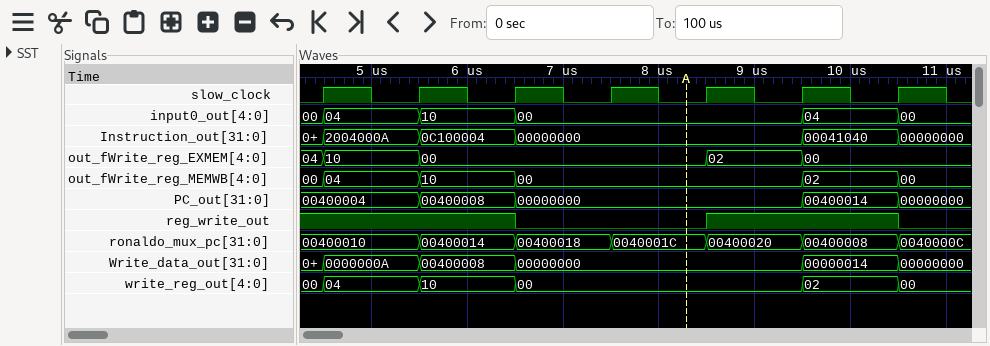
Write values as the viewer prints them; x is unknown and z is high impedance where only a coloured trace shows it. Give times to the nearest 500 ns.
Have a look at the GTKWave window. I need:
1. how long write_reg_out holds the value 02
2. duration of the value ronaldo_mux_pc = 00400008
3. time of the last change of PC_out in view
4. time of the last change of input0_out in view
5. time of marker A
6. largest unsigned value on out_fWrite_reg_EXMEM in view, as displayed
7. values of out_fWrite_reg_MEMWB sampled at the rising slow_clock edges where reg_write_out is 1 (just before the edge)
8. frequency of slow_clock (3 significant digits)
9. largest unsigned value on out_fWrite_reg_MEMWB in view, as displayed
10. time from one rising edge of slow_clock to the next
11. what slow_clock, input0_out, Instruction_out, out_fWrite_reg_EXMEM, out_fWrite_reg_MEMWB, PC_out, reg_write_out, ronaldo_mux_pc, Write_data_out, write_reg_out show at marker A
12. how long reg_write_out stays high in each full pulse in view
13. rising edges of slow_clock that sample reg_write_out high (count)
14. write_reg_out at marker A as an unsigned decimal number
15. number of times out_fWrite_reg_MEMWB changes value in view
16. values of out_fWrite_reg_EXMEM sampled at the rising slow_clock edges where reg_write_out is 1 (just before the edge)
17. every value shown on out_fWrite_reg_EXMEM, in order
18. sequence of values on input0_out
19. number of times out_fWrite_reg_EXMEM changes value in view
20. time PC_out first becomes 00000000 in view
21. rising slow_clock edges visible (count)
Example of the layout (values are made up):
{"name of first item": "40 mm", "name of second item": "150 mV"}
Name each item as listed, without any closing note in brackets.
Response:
{"how long write_reg_out holds the value 02": "1000 ns", "duration of the value ronaldo_mux_pc = 00400008": "1000 ns", "time of the last change of PC_out in view": "10500 ns", "time of the last change of input0_out in view": "10500 ns", "time of marker A": "8500 ns", "largest unsigned value on out_fWrite_reg_EXMEM in view, as displayed": "10", "values of out_fWrite_reg_MEMWB sampled at the rising slow_clock edges where reg_write_out is 1": "00, 04, 10, 00, 02", "frequency of slow_clock": "1.00 MHz", "largest unsigned value on out_fWrite_reg_MEMWB in view, as displayed": "10", "time from one rising edge of slow_clock to the next": "1000 ns", "what slow_clock, input0_out, Instruction_out, out_fWrite_reg_EXMEM, out_fWrite_reg_MEMWB, PC_out, reg_write_out, ronaldo_mux_pc, Write_data_out, write_reg_out show at marker A": "slow_clock=0, input0_out=00, Instruction_out=00000000, out_fWrite_reg_EXMEM=00, out_fWrite_reg_MEMWB=00, PC_out=00000000, reg_write_out=0, ronaldo_mux_pc=0040001C, Write_data_out=00000000, write_reg_out=00", "how long reg_write_out stays high in each full pulse in view": "2000 ns", "rising edges of slow_clock that sample reg_write_out high": "5", "write_reg_out at marker A as an unsigned decimal number": "0", "number of times out_fWrite_reg_MEMWB changes value in view": "5", "values of out_fWrite_reg_EXMEM sampled at the rising slow_clock edges where reg_write_out is 1": "04, 10, 00, 02, 00", "every value shown on out_fWrite_reg_EXMEM, in order": "04, 10, 00, 02, 00", "sequence of values on input0_out": "00, 04, 10, 00, 04, 00", "number of times out_fWrite_reg_EXMEM changes value in view": "4", "time PC_out first becomes 00000000 in view": "6500 ns", "rising slow_clock edges visible": "7"}
